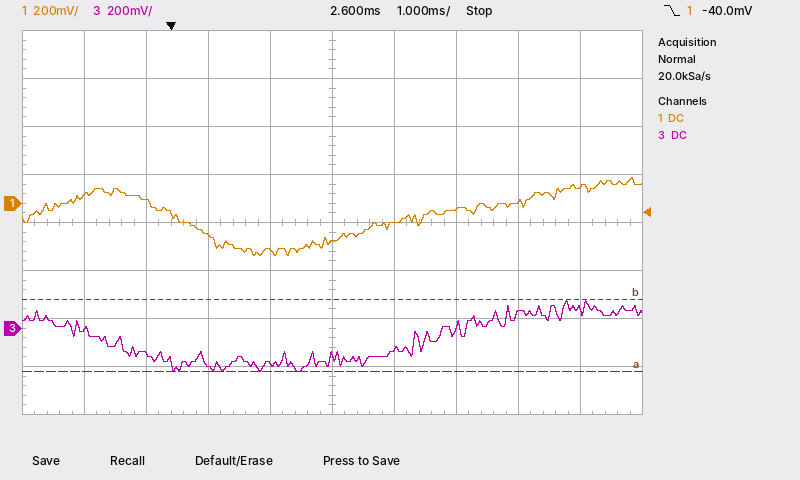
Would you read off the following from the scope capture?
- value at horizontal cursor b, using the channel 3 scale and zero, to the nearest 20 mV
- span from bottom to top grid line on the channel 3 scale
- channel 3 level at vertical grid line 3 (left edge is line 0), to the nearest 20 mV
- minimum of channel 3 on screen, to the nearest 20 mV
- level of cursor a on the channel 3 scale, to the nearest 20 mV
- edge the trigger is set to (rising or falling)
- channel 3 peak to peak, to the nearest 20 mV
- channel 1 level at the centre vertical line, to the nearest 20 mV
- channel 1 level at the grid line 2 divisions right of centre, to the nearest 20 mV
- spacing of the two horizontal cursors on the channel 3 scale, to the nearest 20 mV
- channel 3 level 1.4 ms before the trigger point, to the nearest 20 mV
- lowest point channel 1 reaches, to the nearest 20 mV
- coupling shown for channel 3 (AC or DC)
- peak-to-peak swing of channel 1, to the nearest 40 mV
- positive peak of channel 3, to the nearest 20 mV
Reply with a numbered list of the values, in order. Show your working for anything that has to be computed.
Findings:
1. 120 mV
2. 1.6 V
3. -160 mV
4. -180 mV
5. -180 mV
6. falling
7. 120 mV − (-180 mV) = 300 mV
8. -160 mV
9. -20 mV
10. 300 mV
11. 0 mV
12. -220 mV
13. DC
14. 320 mV
15. 120 mV
